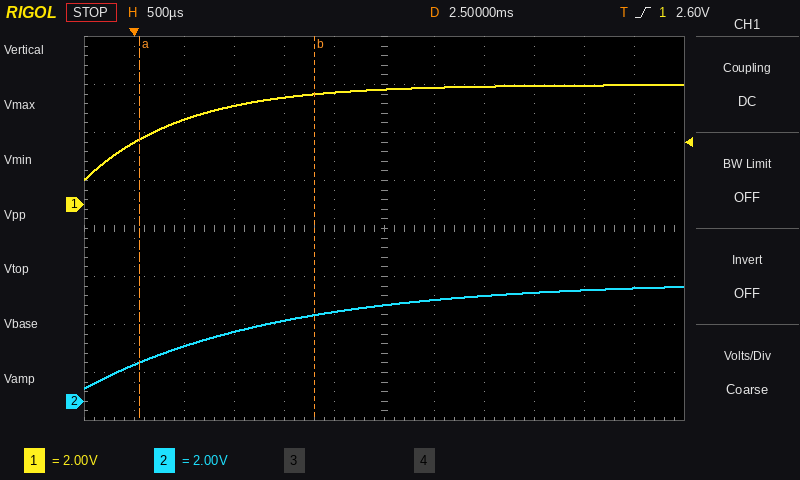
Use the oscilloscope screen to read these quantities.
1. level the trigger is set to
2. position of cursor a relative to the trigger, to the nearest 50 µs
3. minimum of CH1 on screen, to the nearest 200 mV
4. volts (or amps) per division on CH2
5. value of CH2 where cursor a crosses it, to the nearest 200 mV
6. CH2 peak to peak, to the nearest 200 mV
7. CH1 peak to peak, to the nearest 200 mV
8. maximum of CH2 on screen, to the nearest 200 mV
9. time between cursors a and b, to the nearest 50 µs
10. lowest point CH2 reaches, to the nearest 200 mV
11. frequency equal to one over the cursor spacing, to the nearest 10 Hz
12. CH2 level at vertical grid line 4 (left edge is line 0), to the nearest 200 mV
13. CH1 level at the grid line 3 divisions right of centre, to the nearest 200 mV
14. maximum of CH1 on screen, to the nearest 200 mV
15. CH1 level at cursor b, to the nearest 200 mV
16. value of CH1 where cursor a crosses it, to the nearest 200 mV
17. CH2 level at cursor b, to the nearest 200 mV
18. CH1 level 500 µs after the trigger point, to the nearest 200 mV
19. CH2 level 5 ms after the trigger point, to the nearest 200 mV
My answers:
2.60 V
+50 µs
1.0 V
2 V
1.6 V
4.2 V
4.0 V
4.8 V
1.75 ms
600 mV
570 Hz
3.4 V
5.0 V
5.0 V
4.6 V
2.8 V
3.6 V
3.6 V
4.8 V
